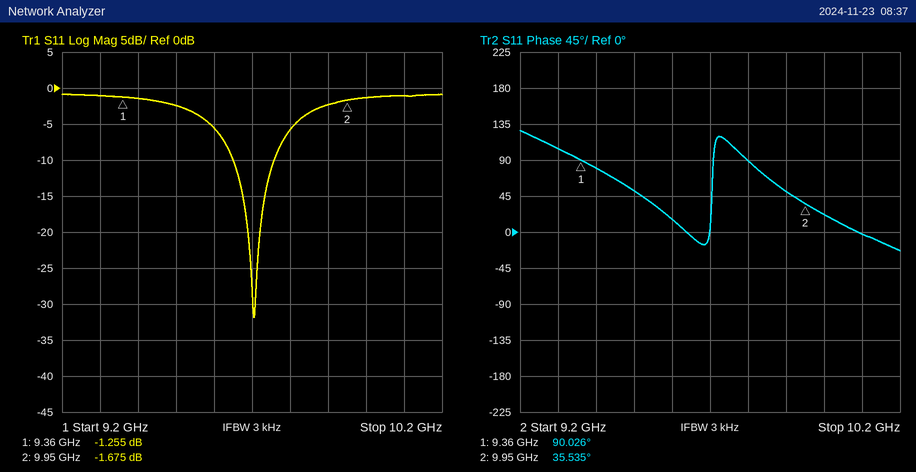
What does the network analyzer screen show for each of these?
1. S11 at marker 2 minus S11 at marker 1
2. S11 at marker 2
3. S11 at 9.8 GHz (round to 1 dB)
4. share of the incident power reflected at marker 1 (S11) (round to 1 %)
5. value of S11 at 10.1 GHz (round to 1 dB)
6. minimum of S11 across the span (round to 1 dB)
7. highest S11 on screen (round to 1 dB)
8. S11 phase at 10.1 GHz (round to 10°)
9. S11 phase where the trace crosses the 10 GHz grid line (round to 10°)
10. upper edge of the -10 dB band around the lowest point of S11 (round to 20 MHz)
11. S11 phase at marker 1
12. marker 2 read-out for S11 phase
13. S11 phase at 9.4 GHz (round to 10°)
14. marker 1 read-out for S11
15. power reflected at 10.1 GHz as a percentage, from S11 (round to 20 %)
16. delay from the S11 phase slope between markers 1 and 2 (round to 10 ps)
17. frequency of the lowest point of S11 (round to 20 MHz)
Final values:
-0.420 dB
-1.675 dB
-6 dB
75 %
-1 dB
-32 dB
-1 dB
0°
20°
9.76 GHz
90.026°
35.535°
80°
-1.255 dB
80 %
260 ps
9.70 GHz
